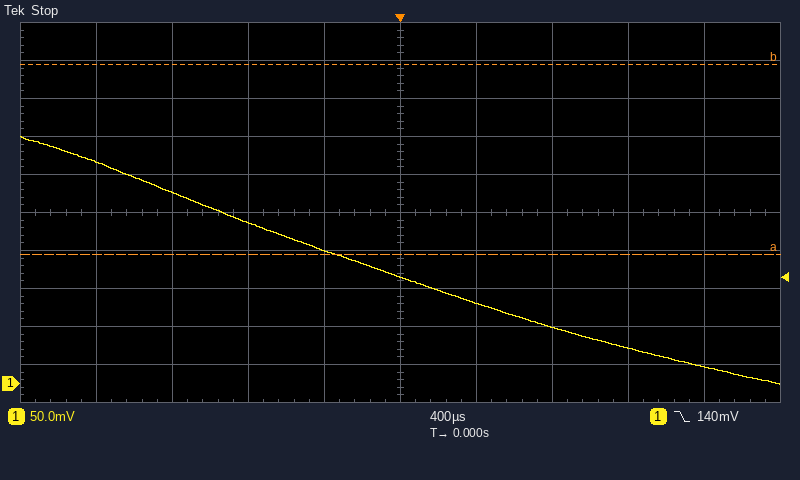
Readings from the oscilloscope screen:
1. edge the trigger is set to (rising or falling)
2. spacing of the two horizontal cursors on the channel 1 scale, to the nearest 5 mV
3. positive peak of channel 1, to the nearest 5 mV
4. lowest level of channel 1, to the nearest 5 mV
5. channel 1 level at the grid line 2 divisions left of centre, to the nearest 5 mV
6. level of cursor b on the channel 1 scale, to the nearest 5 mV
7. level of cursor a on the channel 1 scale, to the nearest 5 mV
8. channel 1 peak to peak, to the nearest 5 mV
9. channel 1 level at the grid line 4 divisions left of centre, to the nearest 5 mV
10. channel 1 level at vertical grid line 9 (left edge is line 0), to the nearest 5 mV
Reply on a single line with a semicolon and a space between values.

falling; 250 mV; 325 mV; 0 mV; 210 mV; 420 mV; 170 mV; 325 mV; 290 mV; 20 mV
